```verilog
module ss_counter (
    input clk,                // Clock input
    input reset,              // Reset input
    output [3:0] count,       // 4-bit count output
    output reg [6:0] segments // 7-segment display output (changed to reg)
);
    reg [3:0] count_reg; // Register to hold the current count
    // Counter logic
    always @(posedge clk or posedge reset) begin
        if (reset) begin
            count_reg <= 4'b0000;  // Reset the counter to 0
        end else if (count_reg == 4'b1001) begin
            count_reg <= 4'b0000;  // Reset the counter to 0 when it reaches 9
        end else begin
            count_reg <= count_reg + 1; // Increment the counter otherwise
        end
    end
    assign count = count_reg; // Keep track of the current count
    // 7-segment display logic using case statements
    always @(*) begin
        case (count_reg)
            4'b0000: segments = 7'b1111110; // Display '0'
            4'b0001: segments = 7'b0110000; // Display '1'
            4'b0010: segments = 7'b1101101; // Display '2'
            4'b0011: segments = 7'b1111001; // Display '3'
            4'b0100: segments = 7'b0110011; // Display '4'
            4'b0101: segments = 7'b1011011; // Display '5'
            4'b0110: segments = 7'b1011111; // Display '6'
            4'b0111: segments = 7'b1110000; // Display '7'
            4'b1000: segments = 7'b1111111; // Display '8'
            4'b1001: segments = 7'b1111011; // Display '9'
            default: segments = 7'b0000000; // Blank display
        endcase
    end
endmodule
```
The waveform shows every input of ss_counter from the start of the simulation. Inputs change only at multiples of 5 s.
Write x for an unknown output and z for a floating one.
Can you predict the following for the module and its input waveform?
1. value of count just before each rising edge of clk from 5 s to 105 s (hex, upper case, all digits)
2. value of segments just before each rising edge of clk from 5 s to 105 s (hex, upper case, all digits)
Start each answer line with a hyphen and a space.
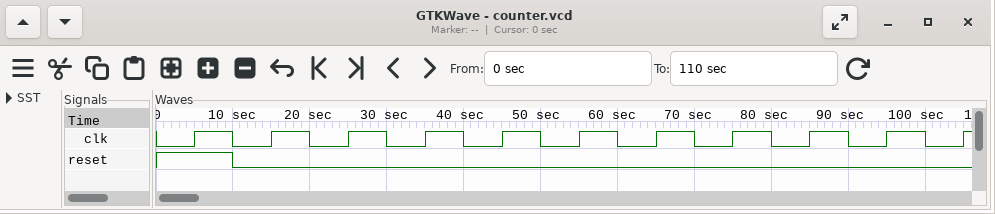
- 0, 0, 1, 2, 3, 4, 5, 6, 7, 8, 9
- 7E, 7E, 30, 6D, 79, 33, 5B, 5F, 70, 7F, 7B
